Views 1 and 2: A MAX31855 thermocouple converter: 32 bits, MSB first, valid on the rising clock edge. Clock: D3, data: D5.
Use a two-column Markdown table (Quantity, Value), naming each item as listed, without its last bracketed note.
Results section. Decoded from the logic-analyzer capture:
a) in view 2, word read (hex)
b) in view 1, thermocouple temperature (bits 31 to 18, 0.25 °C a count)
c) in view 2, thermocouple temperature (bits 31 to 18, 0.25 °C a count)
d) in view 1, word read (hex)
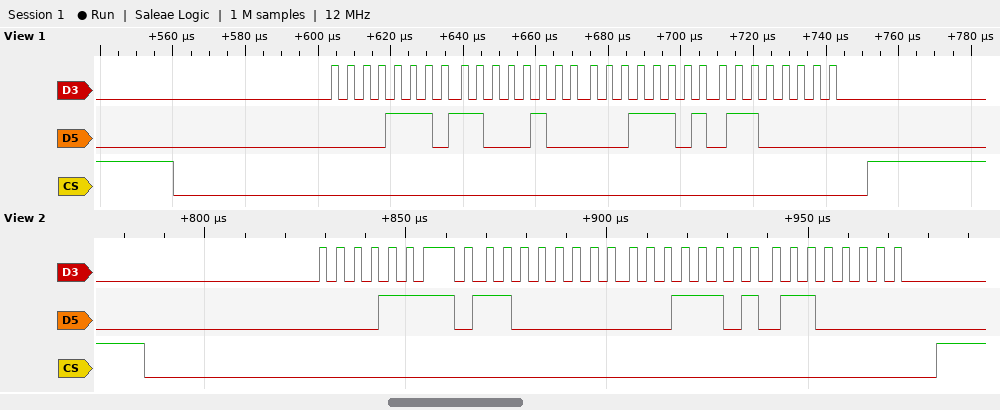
| Quantity | Value |
|---|---|
| in view 2, word read | 0x0EC01D60 |
| in view 1, thermocouple temperature | 236.25 °C |
| in view 2, thermocouple temperature | 236.00 °C |
| in view 1, word read | 0x0EC41D60 |
